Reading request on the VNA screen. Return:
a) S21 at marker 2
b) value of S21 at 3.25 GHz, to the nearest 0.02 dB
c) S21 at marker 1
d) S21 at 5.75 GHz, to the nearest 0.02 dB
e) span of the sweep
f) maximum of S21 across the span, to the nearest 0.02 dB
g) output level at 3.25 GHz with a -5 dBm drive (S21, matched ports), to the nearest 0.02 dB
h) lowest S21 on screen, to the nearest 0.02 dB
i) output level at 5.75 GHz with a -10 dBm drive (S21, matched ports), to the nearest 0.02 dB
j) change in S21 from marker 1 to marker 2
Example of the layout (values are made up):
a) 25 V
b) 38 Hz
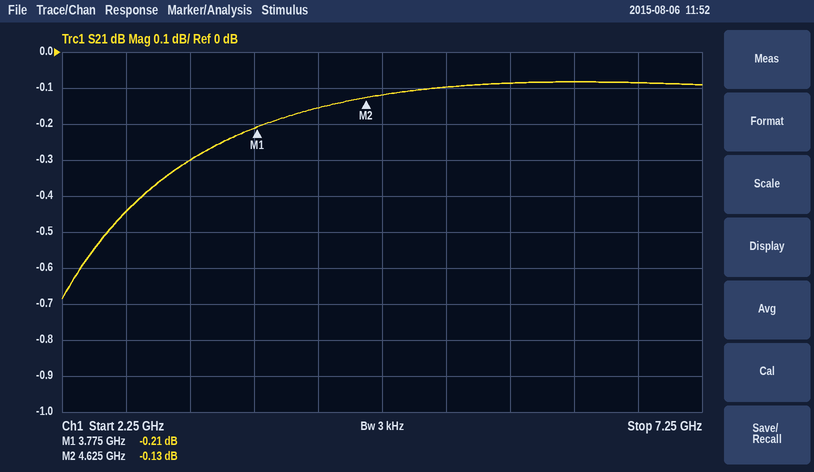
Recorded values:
a) -0.13 dB
b) -0.30 dB
c) -0.21 dB
d) -0.08 dB
e) 5 GHz
f) -0.08 dB
g) -5.30 dBm
h) -0.68 dB
i) -10.08 dBm
j) 0.08 dB
